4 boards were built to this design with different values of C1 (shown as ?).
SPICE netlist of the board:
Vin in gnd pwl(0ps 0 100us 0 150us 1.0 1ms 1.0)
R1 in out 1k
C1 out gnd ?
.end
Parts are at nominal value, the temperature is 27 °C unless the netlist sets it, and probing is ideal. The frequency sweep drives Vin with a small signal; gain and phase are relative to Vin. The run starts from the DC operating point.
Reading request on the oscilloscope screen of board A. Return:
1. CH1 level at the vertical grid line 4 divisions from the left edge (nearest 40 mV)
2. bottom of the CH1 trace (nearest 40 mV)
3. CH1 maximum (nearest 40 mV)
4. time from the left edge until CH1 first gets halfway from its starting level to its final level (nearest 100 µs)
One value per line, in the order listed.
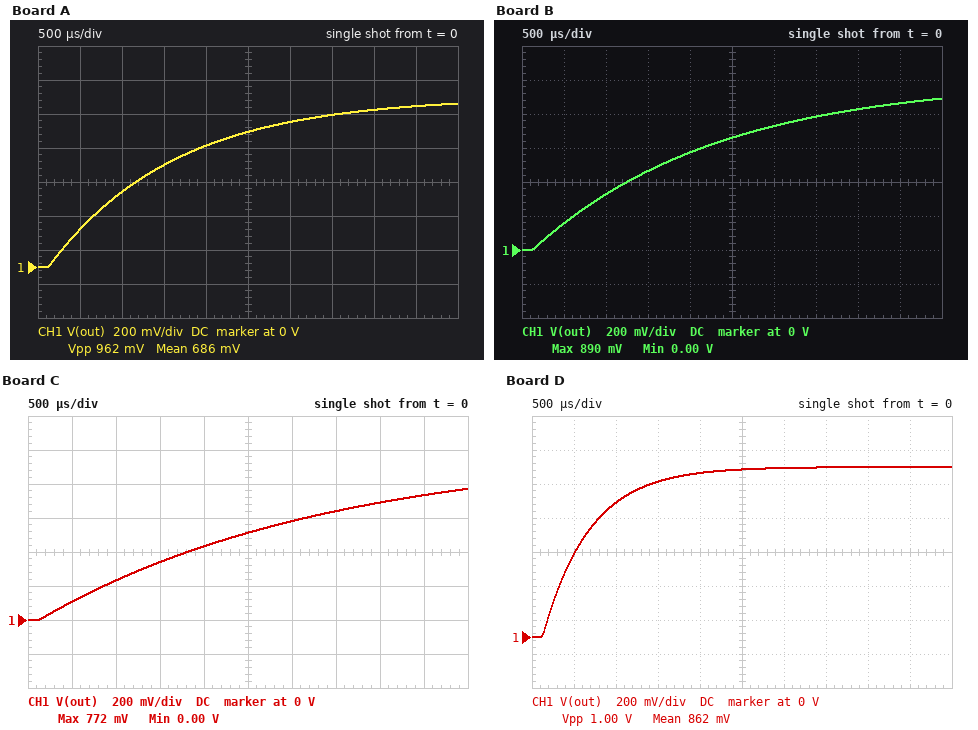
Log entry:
720 mV
0 V
960 mV
1.1 ms
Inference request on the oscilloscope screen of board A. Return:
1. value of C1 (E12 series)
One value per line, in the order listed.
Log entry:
1.5 µF
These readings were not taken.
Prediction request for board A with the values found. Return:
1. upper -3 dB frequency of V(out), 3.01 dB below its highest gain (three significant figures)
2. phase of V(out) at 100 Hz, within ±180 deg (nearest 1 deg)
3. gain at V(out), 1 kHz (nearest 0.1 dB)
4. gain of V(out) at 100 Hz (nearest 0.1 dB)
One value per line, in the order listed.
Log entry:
106 Hz
-43 deg
-19.5 dB
-2.8 dB
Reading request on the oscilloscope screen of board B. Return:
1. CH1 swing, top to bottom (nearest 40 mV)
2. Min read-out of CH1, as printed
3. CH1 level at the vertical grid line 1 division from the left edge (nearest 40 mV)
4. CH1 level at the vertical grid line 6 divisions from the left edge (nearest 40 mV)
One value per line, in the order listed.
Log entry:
880 mV
0.00 V
160 mV
720 mV
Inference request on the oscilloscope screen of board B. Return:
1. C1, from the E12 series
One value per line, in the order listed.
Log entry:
2.2 µF
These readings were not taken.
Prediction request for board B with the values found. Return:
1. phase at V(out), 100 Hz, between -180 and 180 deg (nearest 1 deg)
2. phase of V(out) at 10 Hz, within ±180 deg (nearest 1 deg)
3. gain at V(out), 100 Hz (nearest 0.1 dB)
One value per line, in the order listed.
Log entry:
-54 deg
-8 deg
-4.6 dB
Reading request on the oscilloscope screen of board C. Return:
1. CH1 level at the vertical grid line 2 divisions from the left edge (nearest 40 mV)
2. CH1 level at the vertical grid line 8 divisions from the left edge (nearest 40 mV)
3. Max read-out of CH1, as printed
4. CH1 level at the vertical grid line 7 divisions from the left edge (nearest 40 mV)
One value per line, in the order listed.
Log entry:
240 mV
680 mV
772 mV
640 mV
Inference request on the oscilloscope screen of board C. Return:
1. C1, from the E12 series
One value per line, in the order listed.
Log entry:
3.3 µF
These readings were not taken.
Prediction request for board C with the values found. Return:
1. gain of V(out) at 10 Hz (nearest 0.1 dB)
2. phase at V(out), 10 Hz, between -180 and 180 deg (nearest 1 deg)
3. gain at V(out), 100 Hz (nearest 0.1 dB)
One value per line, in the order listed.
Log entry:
-0.2 dB
-12 deg
-7.2 dB
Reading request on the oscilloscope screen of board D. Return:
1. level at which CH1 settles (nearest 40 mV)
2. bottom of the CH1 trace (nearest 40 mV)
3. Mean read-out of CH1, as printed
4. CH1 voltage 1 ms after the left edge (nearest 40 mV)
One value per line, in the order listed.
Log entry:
1.00 V
0 V
862 mV
800 mV
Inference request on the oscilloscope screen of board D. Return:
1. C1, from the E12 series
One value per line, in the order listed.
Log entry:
560 nF
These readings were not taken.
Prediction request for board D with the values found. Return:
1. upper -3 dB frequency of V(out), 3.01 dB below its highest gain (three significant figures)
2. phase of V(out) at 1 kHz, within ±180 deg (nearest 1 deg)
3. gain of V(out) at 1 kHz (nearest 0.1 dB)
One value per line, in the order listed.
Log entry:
284 Hz
-74 deg
-11.3 dB
